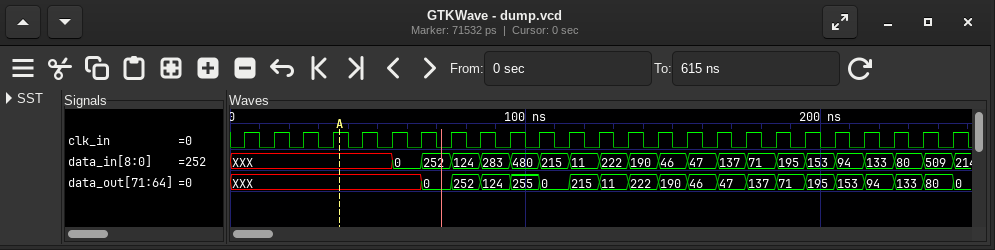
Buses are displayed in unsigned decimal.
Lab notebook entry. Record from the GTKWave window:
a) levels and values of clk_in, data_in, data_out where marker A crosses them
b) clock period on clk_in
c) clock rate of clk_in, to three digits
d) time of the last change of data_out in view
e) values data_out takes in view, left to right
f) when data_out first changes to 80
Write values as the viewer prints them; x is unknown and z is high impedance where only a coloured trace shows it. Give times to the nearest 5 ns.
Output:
clk_in=1, data_in=XXX, data_out=XXX
10 ns
100 MHz
245 ns
XXX, 0, 252, 124, 255, 0, 215, 11, 222, 190, 46, 47, 137, 71, 195, 153, 94, 133, 80, 0
235 ns
